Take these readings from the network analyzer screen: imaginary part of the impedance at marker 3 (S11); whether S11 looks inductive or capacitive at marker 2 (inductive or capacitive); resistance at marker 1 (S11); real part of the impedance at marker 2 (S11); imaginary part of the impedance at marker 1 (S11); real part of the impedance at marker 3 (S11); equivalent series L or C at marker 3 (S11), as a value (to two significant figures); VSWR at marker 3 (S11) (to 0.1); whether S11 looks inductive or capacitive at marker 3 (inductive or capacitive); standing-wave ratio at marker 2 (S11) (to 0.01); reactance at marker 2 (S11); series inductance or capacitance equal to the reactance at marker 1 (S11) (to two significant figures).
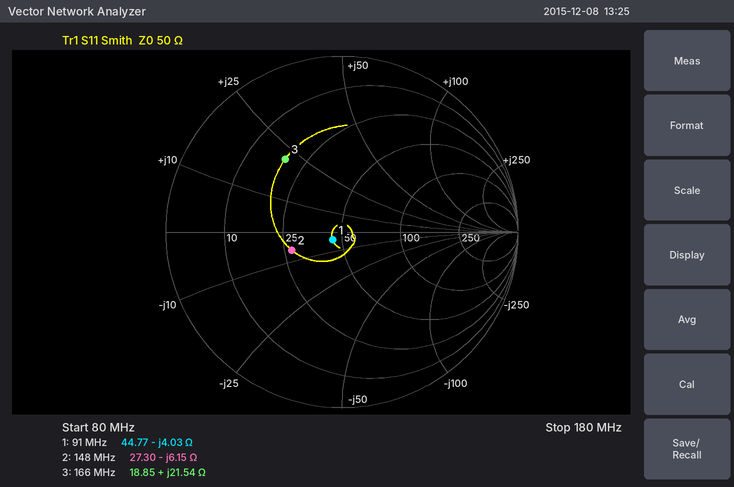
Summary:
+21.54 Ω
capacitive
44.77 Ω
27.30 Ω
-4.03 Ω
18.85 Ω
21 nH
3.2
inductive
1.87
-6.15 Ω
430 pF
